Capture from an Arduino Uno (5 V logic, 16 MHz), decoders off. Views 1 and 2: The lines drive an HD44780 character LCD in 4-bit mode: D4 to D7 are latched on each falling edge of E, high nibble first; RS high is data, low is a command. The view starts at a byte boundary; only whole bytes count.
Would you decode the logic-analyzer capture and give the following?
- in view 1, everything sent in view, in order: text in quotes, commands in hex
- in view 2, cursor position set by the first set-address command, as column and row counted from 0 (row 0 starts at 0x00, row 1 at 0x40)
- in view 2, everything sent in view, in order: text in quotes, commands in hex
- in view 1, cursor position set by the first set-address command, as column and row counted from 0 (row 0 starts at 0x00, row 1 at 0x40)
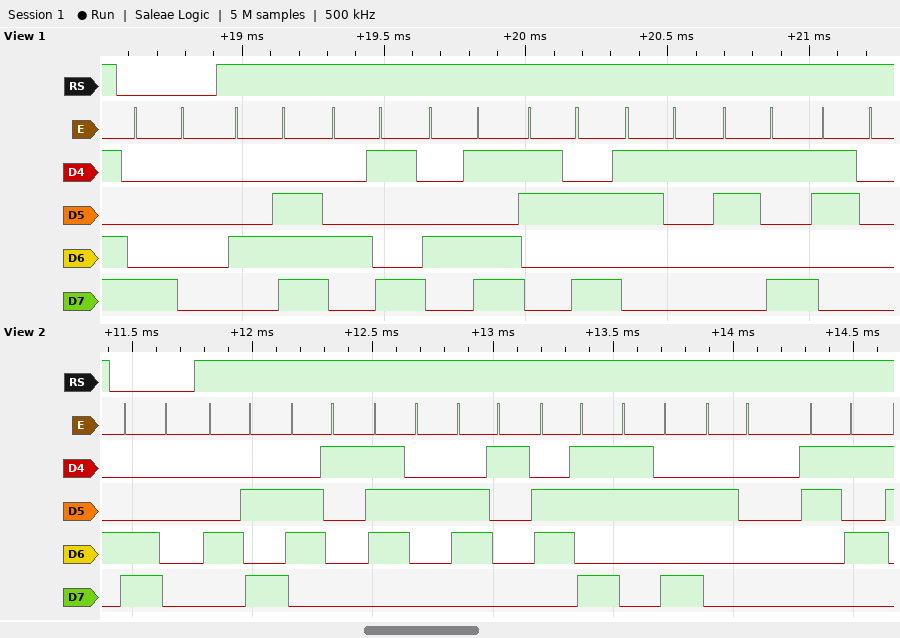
0x80 "NIM:190"
column 0, row 1
0xC0 "Jarak: 5"
column 0, row 0
